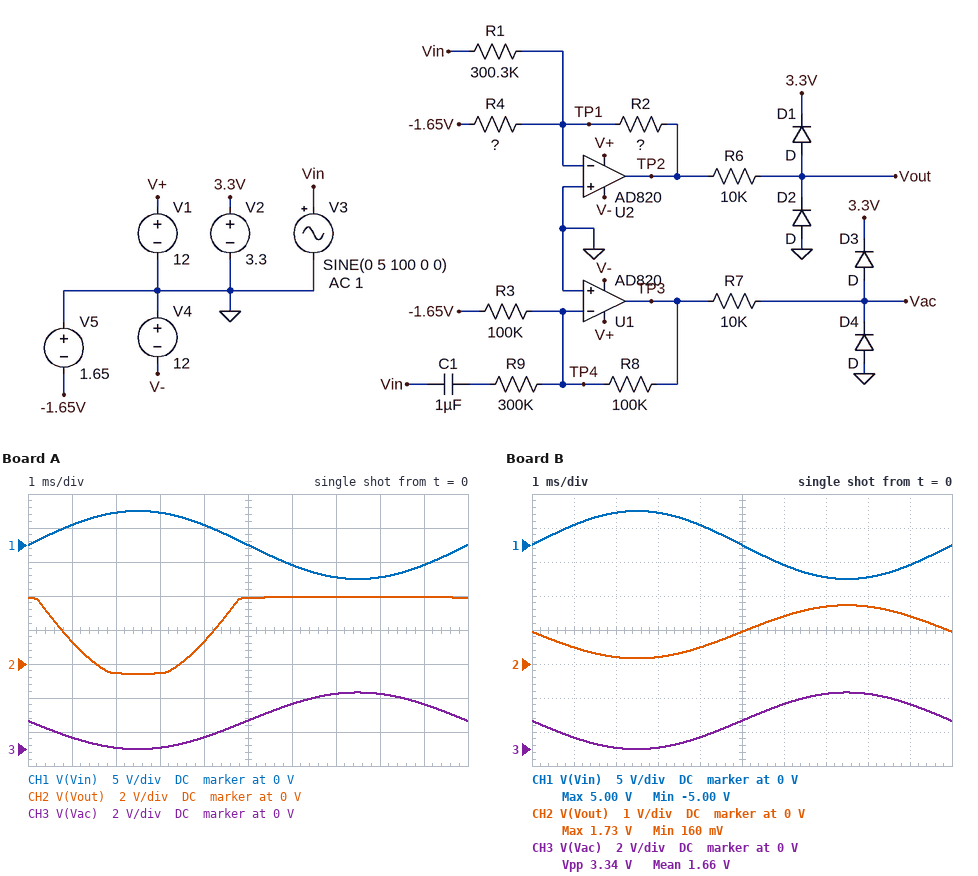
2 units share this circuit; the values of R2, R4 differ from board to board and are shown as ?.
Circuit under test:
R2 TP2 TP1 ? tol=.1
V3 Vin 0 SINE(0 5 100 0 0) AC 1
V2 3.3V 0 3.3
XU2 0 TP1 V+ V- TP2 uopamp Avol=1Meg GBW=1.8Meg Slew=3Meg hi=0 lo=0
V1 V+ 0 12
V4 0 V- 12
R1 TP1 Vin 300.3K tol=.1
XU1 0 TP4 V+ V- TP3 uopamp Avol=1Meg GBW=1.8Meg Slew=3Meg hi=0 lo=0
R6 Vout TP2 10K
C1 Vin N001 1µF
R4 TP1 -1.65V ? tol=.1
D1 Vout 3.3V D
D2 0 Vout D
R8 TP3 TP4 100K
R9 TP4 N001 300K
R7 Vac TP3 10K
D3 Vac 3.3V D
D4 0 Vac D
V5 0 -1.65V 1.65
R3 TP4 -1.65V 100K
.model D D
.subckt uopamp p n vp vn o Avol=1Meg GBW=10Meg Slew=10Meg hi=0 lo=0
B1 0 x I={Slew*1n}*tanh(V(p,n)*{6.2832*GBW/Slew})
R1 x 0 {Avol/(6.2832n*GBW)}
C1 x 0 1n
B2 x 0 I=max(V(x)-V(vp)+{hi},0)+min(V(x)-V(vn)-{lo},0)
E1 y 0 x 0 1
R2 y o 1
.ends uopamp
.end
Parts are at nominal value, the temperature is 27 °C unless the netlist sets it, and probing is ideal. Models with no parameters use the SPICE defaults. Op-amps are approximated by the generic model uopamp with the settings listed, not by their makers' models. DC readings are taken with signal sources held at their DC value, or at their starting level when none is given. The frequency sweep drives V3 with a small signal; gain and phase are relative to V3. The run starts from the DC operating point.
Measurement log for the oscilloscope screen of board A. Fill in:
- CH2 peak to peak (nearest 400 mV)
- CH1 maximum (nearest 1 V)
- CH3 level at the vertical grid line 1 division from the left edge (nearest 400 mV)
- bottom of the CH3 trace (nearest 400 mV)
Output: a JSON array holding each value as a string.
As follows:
["4.4 V", "5 V", "800 mV", "0 V"]
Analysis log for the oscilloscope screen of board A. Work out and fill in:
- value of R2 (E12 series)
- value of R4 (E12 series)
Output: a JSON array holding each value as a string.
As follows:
["330 kΩ", "120 kΩ"]
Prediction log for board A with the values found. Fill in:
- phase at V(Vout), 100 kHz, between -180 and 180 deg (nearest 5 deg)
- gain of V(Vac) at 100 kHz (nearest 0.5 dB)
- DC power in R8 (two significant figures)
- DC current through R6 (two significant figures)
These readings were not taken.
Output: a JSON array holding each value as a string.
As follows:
["165 deg", "-9.5 dB", "27 µW", "65 µA"]
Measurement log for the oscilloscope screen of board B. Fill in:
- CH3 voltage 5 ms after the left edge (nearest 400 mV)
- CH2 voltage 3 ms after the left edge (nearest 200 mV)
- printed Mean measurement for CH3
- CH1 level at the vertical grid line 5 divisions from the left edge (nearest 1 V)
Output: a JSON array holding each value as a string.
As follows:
["1.6 V", "200 mV", "1.66 V", "0 V"]
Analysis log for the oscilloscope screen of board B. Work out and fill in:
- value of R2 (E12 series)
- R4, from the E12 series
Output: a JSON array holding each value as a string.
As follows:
["47 kΩ", "82 kΩ"]
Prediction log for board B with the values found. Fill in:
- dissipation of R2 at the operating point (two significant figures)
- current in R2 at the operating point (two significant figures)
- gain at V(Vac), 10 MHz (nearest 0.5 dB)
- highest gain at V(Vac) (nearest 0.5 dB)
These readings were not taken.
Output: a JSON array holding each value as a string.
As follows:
["19 µW", "20 µA", "-32.0 dB", "-9.5 dB"]
